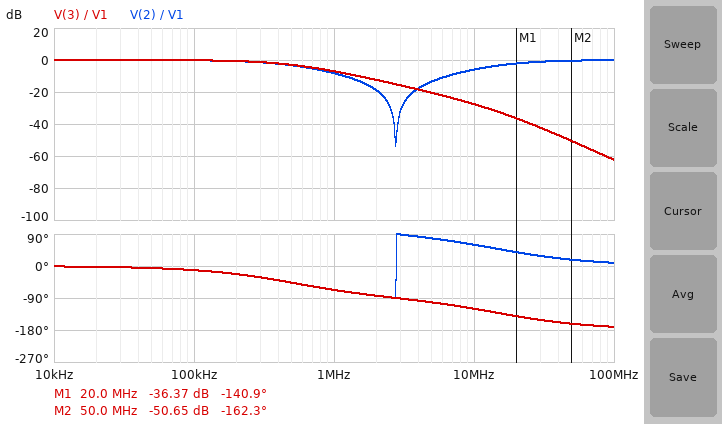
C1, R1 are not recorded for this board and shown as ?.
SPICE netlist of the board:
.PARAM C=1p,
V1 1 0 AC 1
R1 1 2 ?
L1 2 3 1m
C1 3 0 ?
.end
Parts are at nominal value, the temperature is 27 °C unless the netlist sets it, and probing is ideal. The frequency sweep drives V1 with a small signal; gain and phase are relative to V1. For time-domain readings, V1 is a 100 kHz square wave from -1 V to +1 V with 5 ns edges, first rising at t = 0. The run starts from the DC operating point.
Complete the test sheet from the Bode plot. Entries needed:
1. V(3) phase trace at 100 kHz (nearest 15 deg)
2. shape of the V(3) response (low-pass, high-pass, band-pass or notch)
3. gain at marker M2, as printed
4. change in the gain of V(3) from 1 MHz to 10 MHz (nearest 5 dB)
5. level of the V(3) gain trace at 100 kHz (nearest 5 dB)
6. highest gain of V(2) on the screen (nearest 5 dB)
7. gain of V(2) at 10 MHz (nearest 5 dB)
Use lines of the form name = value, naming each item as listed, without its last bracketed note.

V(3) phase trace at 100 kHz = -15 deg
shape of the V(3) response = low-pass
gain at marker M2, as printed = -50.65 dB
change in the gain of V(3) from 1 MHz to 10 MHz = -20 dB
level of the V(3) gain trace at 100 kHz = 0 dB
highest gain of V(2) on the screen = 0 dB
gain of V(2) at 10 MHz = -5 dB
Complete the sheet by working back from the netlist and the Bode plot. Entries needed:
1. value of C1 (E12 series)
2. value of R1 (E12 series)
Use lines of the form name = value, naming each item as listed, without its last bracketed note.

value of C1 = 3.3 pF
value of R1 = 100 kΩ
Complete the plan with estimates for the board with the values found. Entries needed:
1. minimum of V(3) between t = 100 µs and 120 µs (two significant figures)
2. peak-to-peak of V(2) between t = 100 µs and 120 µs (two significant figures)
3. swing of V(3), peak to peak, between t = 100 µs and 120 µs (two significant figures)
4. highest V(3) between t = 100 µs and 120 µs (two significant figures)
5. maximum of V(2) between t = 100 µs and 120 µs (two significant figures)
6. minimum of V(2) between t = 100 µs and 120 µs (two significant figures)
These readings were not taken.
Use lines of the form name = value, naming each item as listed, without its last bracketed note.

minimum of V(3) between t = 100 µs and 120 µs = -1.0 V
peak-to-peak of V(2) between t = 100 µs and 120 µs = 2.0 V
swing of V(3), peak to peak, between t = 100 µs and 120 µs = 2.0 V
highest V(3) between t = 100 µs and 120 µs = 1.0 V
maximum of V(2) between t = 100 µs and 120 µs = 1.0 V
minimum of V(2) between t = 100 µs and 120 µs = -1.0 V
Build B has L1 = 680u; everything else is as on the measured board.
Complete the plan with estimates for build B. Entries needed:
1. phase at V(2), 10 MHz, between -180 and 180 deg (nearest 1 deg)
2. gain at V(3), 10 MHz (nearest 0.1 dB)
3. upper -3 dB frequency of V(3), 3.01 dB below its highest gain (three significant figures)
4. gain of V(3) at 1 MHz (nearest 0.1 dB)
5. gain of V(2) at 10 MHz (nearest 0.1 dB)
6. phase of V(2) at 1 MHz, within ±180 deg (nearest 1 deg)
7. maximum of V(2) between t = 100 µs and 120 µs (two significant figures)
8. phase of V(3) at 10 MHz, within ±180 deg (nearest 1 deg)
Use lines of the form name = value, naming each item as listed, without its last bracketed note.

phase at V(2), 10 MHz, between -180 and 180 deg = 69 deg
gain at V(3), 10 MHz = -26.9 dB
upper -3 dB frequency of V(3), 3.01 dB below its highest gain = 492 kHz
gain of V(3) at 1 MHz = -7.1 dB
gain of V(2) at 10 MHz = -9.0 dB
phase of V(2) at 1 MHz, within ±180 deg = -66 deg
maximum of V(2) between t = 100 µs and 120 µs = 1.0 V
phase of V(3) at 10 MHz, within ±180 deg = -111 deg
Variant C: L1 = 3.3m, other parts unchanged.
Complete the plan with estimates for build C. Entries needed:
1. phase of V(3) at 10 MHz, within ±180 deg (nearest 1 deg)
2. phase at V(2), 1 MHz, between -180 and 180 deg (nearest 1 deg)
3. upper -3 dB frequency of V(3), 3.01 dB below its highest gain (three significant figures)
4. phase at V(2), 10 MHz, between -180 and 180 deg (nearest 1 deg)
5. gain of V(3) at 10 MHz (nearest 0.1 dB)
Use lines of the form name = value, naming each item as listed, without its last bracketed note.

phase of V(3) at 10 MHz, within ±180 deg = -154 deg
phase at V(2), 1 MHz, between -180 and 180 deg = -75 deg
upper -3 dB frequency of V(3), 3.01 dB below its highest gain = 535 kHz
phase at V(2), 10 MHz, between -180 and 180 deg = 26 deg
gain of V(3) at 10 MHz = -33.4 dB
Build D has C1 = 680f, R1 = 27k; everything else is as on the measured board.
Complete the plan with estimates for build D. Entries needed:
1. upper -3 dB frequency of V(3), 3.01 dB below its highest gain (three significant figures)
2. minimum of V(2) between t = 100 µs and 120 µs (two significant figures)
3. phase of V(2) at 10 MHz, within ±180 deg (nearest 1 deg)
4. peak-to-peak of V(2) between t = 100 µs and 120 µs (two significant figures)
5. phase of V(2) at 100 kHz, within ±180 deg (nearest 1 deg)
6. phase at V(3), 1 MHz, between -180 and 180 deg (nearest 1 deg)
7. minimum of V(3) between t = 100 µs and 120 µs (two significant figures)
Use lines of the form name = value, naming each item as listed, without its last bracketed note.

upper -3 dB frequency of V(3), 3.01 dB below its highest gain = 7.25 MHz
minimum of V(2) between t = 100 µs and 120 µs = -1.3 V
phase of V(2) at 10 MHz, within ±180 deg = 34 deg
peak-to-peak of V(2) between t = 100 µs and 120 µs = 2.6 V
phase of V(2) at 100 kHz, within ±180 deg = -1 deg
phase at V(3), 1 MHz, between -180 and 180 deg = -7 deg
minimum of V(3) between t = 100 µs and 120 µs = -1.6 V
